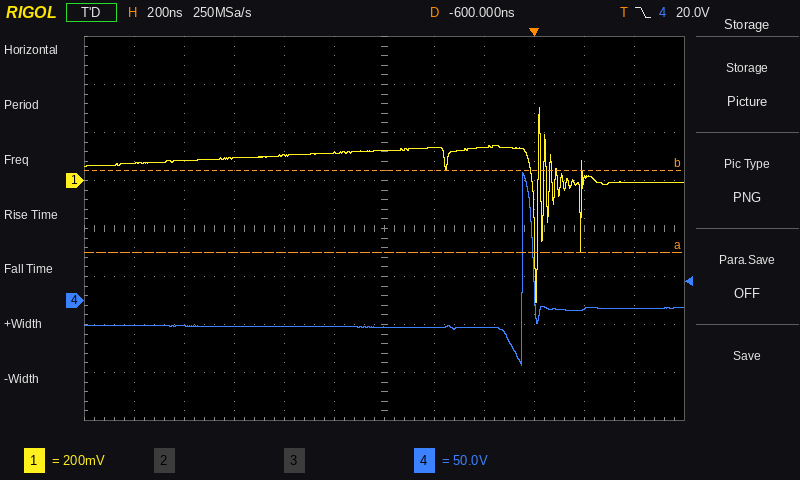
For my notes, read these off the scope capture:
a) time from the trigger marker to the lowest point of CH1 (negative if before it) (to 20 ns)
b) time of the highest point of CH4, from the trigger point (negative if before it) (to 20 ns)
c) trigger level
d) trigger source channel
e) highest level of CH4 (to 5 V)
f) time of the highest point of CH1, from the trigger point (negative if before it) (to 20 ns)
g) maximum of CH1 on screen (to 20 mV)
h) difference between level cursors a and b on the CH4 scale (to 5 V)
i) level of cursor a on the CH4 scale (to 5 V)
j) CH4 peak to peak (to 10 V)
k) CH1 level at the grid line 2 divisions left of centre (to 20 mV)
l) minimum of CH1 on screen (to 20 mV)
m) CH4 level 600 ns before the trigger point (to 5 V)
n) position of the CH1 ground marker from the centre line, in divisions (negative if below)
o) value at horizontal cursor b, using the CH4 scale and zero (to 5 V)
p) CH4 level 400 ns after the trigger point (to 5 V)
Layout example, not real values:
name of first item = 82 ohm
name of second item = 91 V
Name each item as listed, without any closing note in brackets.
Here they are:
time from the trigger marker to the lowest point of CH1 (negative if before it) = 0 ns
time of the highest point of CH4, from the trigger point (negative if before it) = -40 ns
trigger level = 20.0 V
trigger source channel = CH4
highest level of CH4 = 135 V
time of the highest point of CH1, from the trigger point (negative if before it) = +20 ns
maximum of CH1 on screen = 300 mV
difference between level cursors a and b on the CH4 scale = 85 V
level of cursor a on the CH4 scale = 50 V
CH4 peak to peak = 200 V
CH1 level at the grid line 2 divisions left of centre = 100 mV
minimum of CH1 on screen = -500 mV
CH4 level 600 ns before the trigger point = -30 V
position of the CH1 ground marker from the centre line, in divisions = +1.0 div
value at horizontal cursor b, using the CH4 scale and zero = 135 V
CH4 level 400 ns after the trigger point = -10 V
